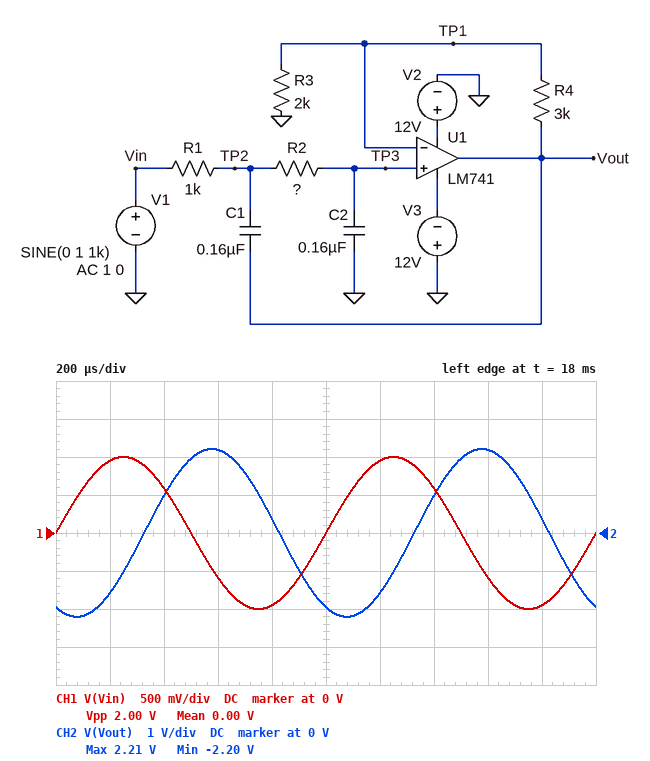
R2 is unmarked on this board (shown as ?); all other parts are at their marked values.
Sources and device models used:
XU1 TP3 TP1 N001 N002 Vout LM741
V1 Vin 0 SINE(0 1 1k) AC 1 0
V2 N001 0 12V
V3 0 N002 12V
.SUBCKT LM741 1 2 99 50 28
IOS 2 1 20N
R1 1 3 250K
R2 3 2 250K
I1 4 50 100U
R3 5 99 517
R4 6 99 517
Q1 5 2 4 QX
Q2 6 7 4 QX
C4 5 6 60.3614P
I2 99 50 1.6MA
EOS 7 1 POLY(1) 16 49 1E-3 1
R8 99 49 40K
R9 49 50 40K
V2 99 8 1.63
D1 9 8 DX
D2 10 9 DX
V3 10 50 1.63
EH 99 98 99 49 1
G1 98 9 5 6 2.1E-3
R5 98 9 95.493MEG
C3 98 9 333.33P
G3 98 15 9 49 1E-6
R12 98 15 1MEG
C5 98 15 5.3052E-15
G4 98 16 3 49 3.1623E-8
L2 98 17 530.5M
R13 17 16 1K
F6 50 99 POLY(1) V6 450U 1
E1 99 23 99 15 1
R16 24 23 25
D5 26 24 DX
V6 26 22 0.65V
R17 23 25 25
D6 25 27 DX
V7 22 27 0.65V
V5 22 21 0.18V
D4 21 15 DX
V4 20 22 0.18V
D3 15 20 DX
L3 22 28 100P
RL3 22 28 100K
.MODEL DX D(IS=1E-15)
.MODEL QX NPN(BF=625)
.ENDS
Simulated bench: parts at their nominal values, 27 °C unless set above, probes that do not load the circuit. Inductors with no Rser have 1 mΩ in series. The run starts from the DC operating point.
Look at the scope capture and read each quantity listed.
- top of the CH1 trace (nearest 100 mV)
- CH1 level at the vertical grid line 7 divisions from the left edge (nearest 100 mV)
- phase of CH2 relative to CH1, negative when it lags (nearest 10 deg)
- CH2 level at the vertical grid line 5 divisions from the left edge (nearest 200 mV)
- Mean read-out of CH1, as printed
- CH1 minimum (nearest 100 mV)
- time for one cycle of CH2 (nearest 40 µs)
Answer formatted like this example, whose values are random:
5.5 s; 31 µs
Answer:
1.0 V; 600 mV; -120 deg; -2.0 V; 0.00 V; -1.0 V; 1.00 ms
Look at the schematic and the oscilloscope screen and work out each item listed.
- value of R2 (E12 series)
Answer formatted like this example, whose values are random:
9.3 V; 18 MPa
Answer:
1.5 kΩ
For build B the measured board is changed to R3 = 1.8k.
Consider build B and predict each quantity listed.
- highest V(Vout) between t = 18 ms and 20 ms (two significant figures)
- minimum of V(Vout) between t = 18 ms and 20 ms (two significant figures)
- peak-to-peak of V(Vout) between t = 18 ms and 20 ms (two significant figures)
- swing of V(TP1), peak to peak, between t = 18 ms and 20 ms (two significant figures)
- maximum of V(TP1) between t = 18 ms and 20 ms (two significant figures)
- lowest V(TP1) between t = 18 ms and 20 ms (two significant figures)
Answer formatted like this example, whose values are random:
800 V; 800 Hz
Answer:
2.7 V; -2.7 V; 5.4 V; 2.0 V; 1.0 V; -1.0 V
